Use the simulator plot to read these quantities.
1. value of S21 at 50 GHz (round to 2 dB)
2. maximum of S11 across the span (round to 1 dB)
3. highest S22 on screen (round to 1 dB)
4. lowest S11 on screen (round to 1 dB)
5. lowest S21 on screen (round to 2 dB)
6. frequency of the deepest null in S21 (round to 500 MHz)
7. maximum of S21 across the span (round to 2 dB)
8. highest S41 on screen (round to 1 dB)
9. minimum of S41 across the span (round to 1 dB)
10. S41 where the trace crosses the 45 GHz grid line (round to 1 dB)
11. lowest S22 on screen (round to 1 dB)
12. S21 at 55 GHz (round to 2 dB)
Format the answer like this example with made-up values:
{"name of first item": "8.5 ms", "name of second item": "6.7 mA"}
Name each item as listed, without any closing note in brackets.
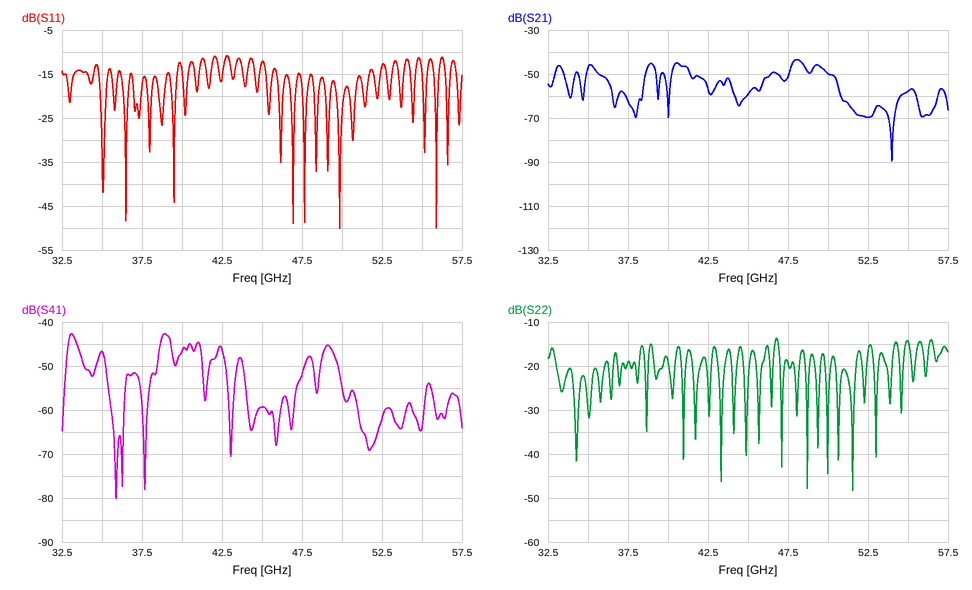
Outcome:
{"value of S21 at 50 GHz": "-50 dB", "maximum of S11 across the span": "-11 dB", "highest S22 on screen": "-14 dB", "lowest S11 on screen": "-50 dB", "lowest S21 on screen": "-90 dB", "frequency of the deepest null in S21": "54.0 GHz", "maximum of S21 across the span": "-44 dB", "highest S41 on screen": "-43 dB", "minimum of S41 across the span": "-80 dB", "S41 where the trace crosses the 45 GHz grid line": "-59 dB", "lowest S22 on screen": "-48 dB", "S21 at 55 GHz": "-58 dB"}
